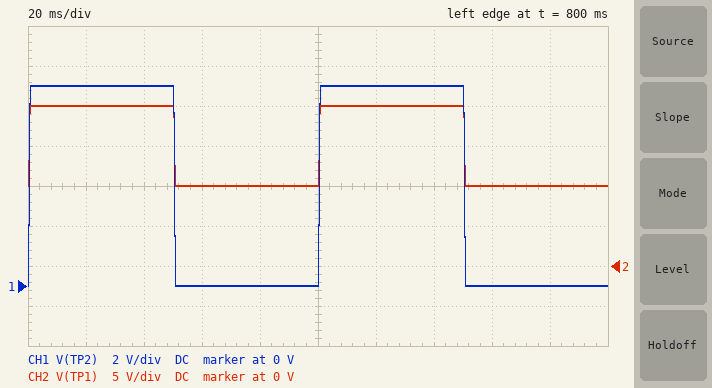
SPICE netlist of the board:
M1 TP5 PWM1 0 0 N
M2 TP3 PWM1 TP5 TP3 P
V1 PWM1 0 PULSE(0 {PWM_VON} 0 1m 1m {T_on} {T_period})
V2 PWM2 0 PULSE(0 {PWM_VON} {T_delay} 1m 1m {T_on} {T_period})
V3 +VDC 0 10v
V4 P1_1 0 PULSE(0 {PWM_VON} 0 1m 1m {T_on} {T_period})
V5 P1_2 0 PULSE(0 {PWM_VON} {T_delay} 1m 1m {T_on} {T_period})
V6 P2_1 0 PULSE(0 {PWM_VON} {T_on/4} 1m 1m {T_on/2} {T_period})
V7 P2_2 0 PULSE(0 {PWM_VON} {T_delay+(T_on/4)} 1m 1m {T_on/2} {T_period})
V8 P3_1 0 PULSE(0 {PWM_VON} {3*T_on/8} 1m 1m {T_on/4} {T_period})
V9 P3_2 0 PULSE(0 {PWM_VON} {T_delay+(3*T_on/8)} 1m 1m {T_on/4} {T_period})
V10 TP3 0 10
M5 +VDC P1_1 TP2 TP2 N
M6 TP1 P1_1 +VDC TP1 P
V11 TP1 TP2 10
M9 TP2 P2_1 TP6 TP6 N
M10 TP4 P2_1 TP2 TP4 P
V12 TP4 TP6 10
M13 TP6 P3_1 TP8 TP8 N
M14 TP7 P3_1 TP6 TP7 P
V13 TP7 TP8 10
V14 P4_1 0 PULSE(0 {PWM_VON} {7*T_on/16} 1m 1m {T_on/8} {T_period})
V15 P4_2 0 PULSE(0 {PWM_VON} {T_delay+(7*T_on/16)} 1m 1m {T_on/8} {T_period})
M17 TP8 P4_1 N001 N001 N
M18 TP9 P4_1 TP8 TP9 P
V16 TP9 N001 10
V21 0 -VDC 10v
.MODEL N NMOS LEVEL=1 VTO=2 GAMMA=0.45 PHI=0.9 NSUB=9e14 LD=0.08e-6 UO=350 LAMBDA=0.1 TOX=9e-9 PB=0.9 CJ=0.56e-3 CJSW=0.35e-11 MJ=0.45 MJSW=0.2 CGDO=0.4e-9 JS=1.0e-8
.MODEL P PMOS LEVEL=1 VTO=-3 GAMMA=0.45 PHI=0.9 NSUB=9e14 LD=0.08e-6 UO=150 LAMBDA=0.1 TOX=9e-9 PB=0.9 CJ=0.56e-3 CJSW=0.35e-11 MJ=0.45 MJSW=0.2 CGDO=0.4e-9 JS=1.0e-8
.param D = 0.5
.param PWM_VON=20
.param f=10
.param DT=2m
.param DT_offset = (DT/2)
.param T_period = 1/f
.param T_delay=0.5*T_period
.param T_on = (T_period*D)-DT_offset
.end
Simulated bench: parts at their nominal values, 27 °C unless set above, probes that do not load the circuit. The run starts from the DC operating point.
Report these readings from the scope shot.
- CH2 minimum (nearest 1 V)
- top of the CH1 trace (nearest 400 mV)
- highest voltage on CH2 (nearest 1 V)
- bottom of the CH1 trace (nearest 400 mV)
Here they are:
10 V
10.0 V
20 V
0 V
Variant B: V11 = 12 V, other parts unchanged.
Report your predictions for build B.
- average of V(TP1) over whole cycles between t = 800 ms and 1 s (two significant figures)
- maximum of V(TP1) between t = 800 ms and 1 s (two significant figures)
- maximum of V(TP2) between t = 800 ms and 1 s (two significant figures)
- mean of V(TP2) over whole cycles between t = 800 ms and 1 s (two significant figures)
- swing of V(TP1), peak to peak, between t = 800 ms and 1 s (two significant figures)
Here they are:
16 V
22 V
10 V
4.0 V
12 V
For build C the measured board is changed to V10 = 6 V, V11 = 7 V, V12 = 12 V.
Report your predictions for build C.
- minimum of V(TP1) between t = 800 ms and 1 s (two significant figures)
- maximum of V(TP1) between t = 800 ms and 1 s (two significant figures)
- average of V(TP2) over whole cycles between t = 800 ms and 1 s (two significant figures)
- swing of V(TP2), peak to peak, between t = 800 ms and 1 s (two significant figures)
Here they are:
10 V
17 V
6.5 V
7.0 V
